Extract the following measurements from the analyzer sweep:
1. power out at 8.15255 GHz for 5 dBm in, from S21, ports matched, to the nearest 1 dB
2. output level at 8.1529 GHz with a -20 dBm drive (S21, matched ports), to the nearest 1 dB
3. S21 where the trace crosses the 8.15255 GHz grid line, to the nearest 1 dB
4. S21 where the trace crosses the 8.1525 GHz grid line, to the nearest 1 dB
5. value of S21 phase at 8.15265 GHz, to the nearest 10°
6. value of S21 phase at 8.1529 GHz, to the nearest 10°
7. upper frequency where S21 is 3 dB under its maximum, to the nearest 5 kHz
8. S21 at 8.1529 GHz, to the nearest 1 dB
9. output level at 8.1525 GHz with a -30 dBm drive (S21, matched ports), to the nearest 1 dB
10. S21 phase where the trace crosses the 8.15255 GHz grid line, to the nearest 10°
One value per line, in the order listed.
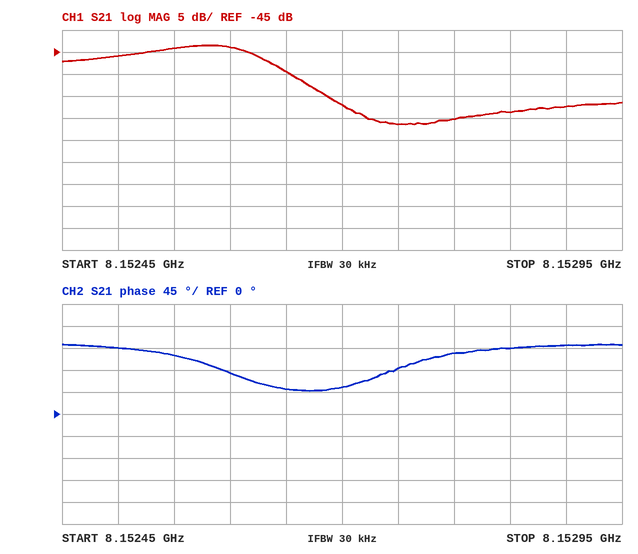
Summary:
-39 dBm
-77 dBm
-44 dB
-46 dB
50°
140°
8.152630 GHz
-57 dB
-76 dBm
120°
